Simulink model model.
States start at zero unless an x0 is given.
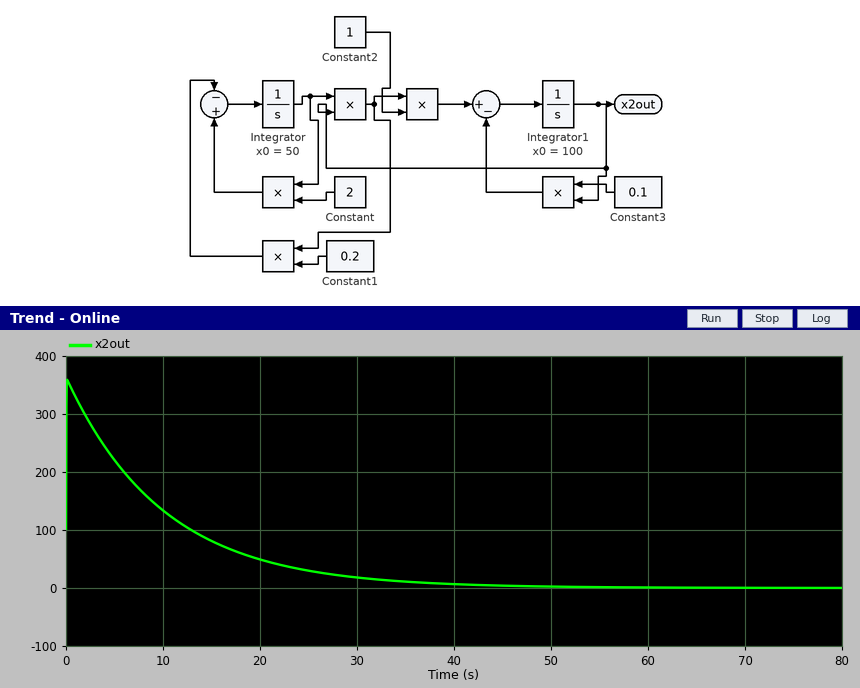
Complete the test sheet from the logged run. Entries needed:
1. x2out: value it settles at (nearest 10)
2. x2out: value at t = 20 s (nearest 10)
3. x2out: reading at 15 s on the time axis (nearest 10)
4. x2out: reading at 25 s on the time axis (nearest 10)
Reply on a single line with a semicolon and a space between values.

0; 50; 80; 30
